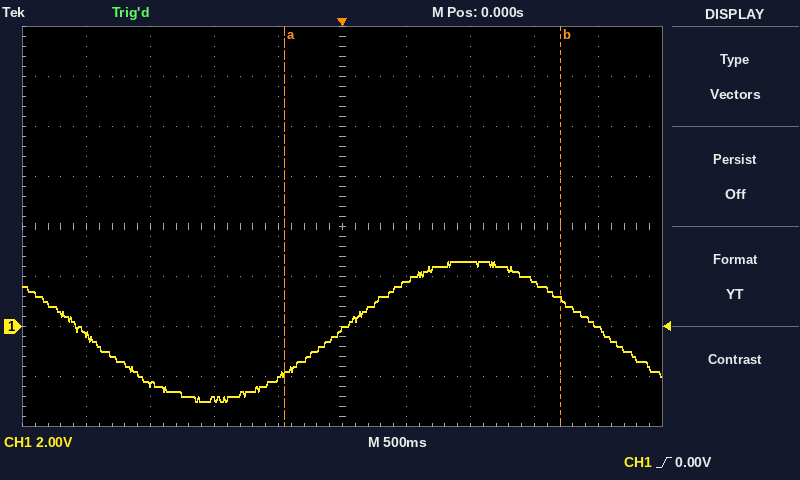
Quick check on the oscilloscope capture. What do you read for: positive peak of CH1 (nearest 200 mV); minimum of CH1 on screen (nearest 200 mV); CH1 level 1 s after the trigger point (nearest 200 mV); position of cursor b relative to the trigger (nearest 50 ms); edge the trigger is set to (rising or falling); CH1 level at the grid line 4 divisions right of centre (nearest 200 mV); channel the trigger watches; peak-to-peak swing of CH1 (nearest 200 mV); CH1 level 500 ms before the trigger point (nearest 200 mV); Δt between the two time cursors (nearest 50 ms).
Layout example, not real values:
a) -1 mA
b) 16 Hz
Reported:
a) 2.6 V
b) -3.0 V
c) 2.6 V
d) +1.70 s
e) rising
f) 0.0 V
g) CH1
h) 5.6 V
i) -2.0 V
j) 2.15 s
